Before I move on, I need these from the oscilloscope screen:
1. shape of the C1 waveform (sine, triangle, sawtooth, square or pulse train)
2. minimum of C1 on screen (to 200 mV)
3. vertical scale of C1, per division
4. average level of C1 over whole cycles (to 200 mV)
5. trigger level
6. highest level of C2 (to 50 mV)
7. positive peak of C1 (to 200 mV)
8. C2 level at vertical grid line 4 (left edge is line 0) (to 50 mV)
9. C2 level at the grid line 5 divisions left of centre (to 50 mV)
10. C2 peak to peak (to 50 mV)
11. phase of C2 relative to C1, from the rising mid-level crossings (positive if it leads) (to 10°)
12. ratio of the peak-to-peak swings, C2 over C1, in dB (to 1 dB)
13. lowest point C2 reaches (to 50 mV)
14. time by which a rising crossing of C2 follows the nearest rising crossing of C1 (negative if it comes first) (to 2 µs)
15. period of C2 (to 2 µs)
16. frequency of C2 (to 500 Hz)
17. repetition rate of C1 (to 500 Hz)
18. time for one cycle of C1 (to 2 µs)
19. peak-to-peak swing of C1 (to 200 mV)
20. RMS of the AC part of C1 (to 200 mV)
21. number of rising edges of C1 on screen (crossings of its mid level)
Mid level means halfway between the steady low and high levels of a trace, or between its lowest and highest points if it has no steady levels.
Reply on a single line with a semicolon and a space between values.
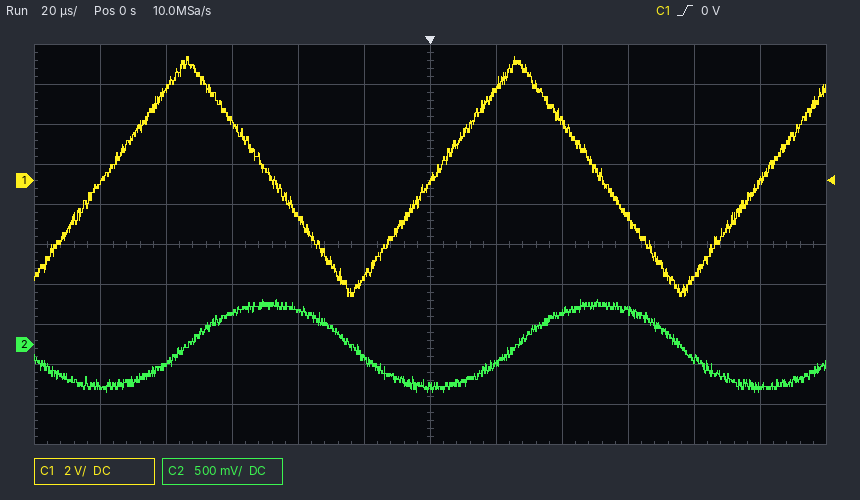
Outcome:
triangle; -5.8 V; 2 V; 200 mV; 0 V; 550 mV; 6.2 V; 400 mV; -500 mV; 1.15 V; -90°; -20 dB; -600 mV; +24 µs; 100 µs; 10.0 kHz; 10.0 kHz; 100 µs; 12.0 V; 3.4 V; 3
